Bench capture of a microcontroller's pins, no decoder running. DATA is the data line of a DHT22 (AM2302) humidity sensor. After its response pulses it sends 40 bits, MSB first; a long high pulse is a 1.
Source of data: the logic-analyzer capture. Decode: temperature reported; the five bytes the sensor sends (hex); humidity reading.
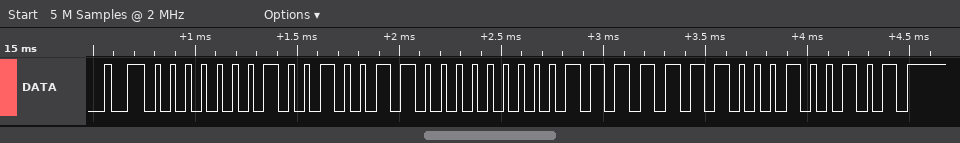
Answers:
25.4 °C
01 26 00 FE 25
29.4 %
